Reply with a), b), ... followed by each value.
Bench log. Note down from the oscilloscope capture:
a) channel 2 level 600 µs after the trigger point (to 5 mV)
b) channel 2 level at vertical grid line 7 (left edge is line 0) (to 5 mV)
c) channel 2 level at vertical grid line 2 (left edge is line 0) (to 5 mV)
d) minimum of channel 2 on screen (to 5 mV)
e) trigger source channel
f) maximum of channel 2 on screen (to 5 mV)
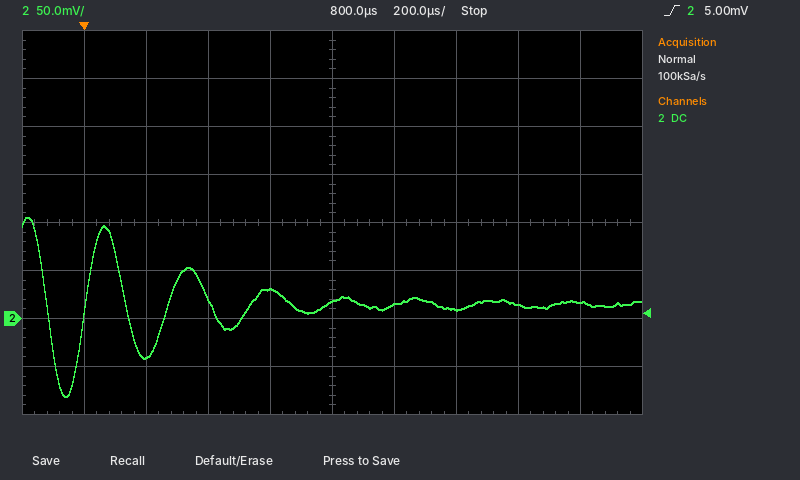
a) 30 mV
b) 10 mV
c) -40 mV
d) -80 mV
e) channel 2
f) 105 mV
